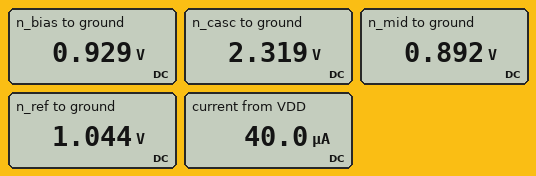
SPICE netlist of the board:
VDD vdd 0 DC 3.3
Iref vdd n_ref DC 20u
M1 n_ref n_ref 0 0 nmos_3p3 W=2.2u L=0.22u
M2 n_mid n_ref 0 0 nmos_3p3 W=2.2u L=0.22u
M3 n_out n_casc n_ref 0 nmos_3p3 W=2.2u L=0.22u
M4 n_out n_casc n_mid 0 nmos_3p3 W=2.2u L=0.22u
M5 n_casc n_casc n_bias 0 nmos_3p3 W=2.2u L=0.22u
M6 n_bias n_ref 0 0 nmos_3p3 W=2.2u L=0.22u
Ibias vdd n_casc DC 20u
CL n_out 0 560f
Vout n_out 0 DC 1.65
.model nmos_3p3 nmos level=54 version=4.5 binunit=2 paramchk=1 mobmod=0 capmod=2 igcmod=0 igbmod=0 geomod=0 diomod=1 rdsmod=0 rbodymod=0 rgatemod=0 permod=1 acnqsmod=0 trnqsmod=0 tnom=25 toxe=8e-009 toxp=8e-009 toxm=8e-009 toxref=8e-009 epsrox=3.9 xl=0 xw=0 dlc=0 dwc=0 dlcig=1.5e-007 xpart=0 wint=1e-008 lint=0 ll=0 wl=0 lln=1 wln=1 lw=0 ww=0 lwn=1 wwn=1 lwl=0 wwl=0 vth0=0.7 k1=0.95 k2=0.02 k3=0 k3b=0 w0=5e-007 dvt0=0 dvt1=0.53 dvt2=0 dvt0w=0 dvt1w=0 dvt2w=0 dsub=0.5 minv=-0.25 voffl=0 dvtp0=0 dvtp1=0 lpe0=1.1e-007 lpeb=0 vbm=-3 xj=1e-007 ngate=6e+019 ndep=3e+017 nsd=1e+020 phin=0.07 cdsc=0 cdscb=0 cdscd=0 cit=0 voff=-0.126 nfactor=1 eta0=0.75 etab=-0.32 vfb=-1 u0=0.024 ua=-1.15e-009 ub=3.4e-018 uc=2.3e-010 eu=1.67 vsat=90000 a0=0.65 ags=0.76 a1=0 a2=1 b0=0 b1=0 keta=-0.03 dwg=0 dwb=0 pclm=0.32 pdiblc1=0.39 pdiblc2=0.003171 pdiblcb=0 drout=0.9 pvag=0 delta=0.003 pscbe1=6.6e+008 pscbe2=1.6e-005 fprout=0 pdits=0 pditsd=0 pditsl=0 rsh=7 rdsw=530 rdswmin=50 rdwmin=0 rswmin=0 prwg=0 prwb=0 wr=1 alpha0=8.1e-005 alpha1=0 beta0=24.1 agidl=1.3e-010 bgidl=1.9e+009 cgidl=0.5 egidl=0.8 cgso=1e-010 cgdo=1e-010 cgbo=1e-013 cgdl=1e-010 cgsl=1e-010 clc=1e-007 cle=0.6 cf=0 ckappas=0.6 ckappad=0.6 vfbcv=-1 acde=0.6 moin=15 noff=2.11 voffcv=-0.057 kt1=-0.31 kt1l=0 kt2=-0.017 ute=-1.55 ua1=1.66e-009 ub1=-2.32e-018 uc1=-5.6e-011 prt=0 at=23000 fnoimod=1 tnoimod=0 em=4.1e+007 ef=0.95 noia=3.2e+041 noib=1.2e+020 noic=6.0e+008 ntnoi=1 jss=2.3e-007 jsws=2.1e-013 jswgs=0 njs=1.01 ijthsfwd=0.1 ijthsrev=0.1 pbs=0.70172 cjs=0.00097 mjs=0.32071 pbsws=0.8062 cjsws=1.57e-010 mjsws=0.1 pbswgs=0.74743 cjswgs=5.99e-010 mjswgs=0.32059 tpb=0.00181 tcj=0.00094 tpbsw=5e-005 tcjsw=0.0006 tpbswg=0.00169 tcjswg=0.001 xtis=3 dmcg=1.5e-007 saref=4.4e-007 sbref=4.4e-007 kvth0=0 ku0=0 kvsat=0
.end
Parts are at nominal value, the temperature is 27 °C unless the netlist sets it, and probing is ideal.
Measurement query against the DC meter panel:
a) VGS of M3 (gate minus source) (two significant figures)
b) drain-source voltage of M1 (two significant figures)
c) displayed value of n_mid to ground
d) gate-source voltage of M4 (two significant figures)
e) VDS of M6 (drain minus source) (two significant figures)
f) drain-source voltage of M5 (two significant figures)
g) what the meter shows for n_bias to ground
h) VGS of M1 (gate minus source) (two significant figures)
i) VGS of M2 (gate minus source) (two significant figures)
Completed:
1.3 V
1.0 V
0.892 V
1.4 V
930 mV
1.4 V
0.929 V
1.0 V
1.0 V
